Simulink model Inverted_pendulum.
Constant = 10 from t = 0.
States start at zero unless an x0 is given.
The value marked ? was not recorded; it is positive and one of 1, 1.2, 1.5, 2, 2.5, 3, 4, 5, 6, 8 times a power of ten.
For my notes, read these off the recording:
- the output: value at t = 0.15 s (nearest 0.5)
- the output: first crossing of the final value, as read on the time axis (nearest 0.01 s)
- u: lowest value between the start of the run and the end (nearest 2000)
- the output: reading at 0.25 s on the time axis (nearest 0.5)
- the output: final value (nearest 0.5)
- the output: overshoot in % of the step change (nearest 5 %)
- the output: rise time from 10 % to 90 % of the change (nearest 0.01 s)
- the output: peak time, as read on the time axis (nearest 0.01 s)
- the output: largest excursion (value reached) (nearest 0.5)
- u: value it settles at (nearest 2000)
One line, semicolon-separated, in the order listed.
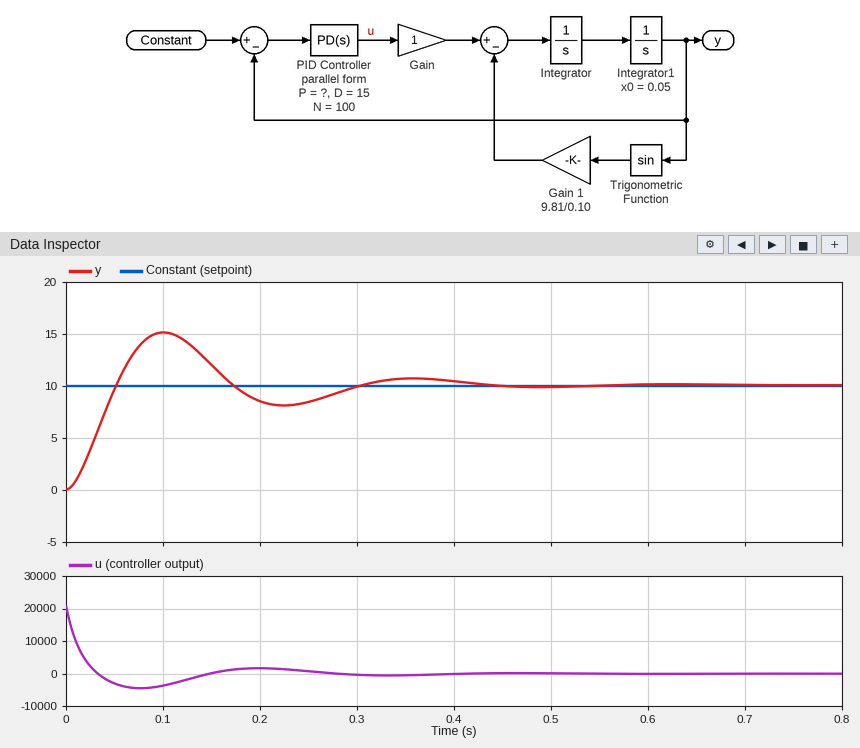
12.0; 0.05 s; -4000; 8.5; 10.0; 50 %; 0.04 s; 0.10 s; 15.0; 0
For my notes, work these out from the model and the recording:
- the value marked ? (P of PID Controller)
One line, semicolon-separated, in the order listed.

600
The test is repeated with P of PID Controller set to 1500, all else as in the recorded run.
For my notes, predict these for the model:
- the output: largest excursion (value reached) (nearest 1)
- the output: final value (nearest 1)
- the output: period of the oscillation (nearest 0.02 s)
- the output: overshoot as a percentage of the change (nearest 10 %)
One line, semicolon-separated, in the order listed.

17; 10; 0.16 s; 70 %
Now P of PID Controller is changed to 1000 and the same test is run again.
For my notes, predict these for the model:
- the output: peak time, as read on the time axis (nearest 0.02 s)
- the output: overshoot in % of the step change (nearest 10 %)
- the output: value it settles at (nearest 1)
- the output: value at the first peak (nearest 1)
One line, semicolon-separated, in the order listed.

0.08 s; 60 %; 10; 16
